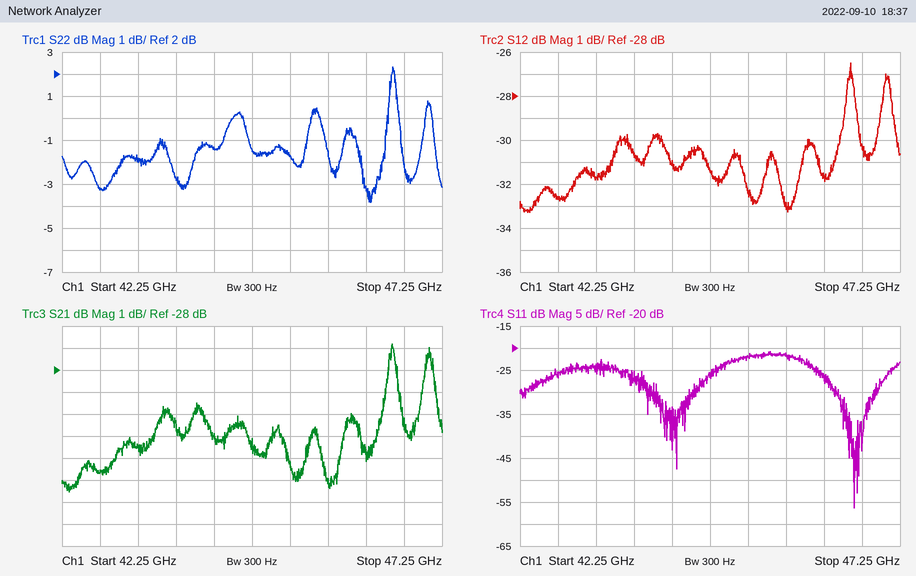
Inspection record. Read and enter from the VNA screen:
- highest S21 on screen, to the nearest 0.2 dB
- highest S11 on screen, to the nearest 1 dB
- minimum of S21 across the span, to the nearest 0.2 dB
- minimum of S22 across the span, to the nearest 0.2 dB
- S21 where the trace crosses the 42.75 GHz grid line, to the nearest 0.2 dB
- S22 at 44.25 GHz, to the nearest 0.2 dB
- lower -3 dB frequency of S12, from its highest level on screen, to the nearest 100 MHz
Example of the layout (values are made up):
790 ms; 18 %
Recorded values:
-26.8 dB; -21 dB; -33.6 dB; -3.8 dB; -32.6 dB; -1.4 dB; 46.5 GHz
